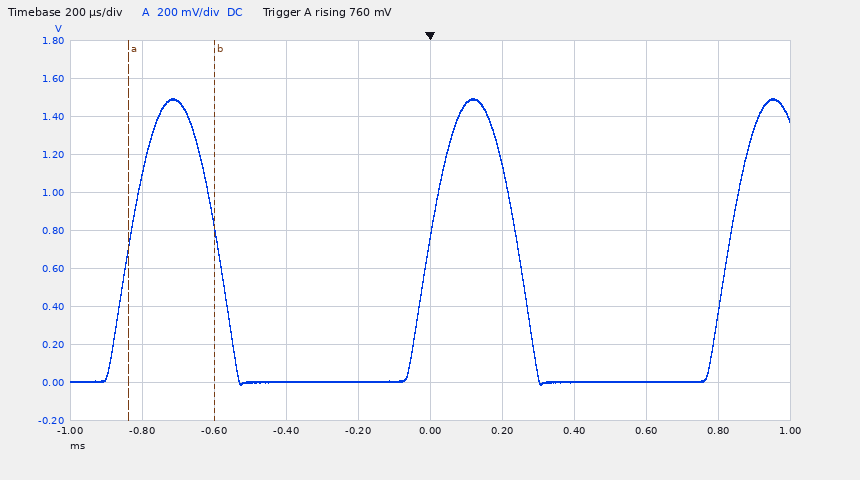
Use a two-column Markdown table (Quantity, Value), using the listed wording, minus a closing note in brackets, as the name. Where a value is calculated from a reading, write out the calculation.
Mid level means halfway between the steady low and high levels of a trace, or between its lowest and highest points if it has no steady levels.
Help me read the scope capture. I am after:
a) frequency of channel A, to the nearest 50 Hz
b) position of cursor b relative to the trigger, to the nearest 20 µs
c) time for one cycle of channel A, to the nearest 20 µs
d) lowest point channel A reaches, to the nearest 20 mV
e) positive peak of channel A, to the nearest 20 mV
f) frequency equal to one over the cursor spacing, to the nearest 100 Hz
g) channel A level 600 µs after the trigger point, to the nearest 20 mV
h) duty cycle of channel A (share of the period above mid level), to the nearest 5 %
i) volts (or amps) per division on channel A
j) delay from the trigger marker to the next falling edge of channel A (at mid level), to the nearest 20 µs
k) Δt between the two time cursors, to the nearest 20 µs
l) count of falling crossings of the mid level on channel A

| Quantity | Value |
|---|---|
| frequency of channel A, to the nearest 50 Hz | 1 / 840 µs ≈ 1.19 kHz, so 1.20 kHz to the nearest 50 Hz |
| position of cursor b relative to the trigger, to the nearest 20 µs | -600 µs |
| time for one cycle of channel A, to the nearest 20 µs | 840 µs |
| lowest point channel A reaches, to the nearest 20 mV | -20 mV |
| positive peak of channel A, to the nearest 20 mV | 1.50 V |
| frequency equal to one over the cursor spacing, to the nearest 100 Hz | 1 / 240 µs ≈ 4.2 kHz |
| channel A level 600 µs after the trigger point, to the nearest 20 mV | 0 mV |
| duty cycle of channel A (share of the period above mid level), to the nearest 5 % | 30 % |
| volts (or amps) per division on channel A | 200 mV |
| delay from the trigger marker to the next falling edge of channel A (at mid level), to the nearest 20 µs | 240 µs |
| Δt between the two time cursors, to the nearest 20 µs | 240 µs |
| count of falling crossings of the mid level on channel A | 2 |
